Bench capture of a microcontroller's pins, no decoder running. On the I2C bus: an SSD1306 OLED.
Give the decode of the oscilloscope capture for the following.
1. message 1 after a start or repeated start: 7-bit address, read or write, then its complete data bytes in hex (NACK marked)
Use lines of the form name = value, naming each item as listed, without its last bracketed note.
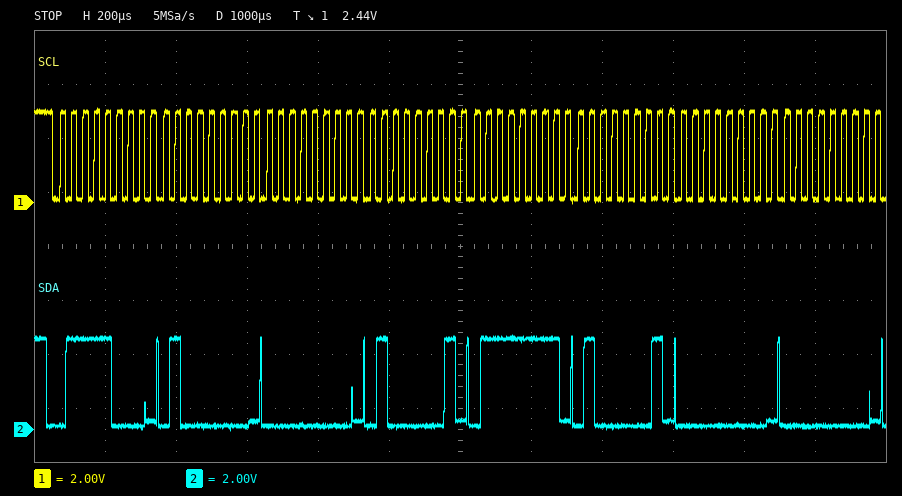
message 1 after a start or repeated start: 7-bit address, read or write, then its complete data bytes in hex = 0x3C write: 40 00 41 7F 41 00 00
